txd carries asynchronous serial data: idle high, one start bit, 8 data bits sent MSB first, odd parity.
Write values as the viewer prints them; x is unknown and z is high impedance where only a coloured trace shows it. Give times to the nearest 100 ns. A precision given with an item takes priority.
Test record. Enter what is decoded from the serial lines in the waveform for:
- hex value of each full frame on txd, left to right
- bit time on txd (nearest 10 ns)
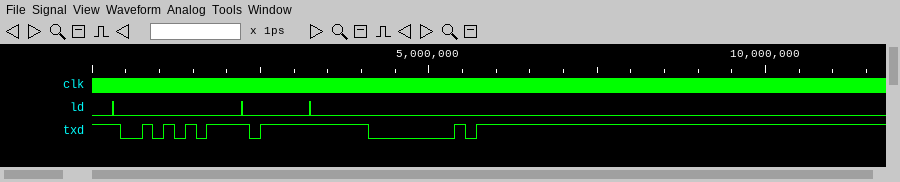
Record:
55, FF, 01
160 ns
